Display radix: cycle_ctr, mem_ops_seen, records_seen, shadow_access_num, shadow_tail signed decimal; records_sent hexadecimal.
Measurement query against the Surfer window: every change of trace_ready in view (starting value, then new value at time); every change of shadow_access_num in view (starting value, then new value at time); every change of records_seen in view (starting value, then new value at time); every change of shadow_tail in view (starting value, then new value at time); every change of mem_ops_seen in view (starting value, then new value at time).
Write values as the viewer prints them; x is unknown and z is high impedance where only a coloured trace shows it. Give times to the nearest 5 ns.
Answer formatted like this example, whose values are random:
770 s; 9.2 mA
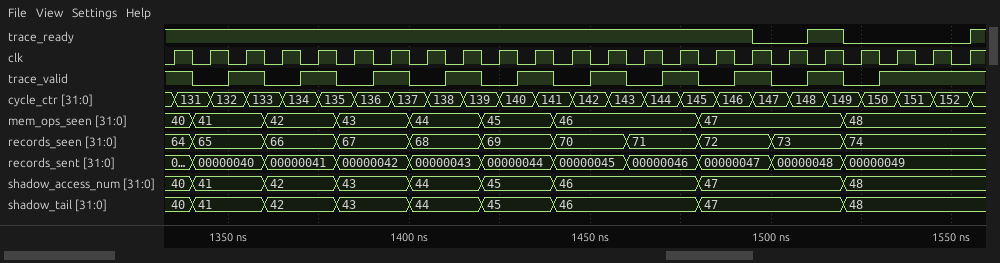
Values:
1, 0 at 1495 ns, 1 at 1510 ns, 0 at 1520 ns, 1 at 1555 ns; 40, 41 at 1340 ns, 42 at 1360 ns, 43 at 1380 ns, 44 at 1400 ns, 45 at 1420 ns, 46 at 1440 ns, 47 at 1480 ns, 48 at 1520 ns; 64, 65 at 1340 ns, 66 at 1360 ns, 67 at 1380 ns, 68 at 1400 ns, 69 at 1420 ns, 70 at 1440 ns, 71 at 1460 ns, 72 at 1480 ns, 73 at 1500 ns, 74 at 1520 ns; 40, 41 at 1340 ns, 42 at 1360 ns, 43 at 1380 ns, 44 at 1400 ns, 45 at 1420 ns, 46 at 1440 ns, 47 at 1480 ns, 48 at 1520 ns; 40, 41 at 1340 ns, 42 at 1360 ns, 43 at 1380 ns, 44 at 1400 ns, 45 at 1420 ns, 46 at 1440 ns, 47 at 1480 ns, 48 at 1520 ns
